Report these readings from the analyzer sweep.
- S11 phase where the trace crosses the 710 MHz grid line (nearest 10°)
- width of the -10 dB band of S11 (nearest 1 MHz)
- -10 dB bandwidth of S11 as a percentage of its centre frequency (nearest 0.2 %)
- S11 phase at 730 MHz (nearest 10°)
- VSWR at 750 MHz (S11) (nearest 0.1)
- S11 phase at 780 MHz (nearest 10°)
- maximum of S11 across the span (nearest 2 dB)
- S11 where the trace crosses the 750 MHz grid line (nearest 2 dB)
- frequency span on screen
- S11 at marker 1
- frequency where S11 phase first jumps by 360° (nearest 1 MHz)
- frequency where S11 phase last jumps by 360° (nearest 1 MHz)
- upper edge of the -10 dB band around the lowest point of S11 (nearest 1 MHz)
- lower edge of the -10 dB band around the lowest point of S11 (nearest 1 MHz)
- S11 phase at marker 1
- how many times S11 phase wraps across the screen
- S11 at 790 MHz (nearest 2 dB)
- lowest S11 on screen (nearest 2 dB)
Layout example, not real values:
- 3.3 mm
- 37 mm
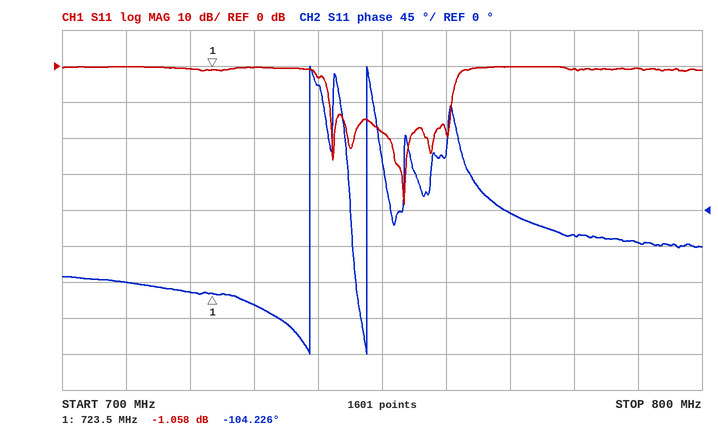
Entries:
- -90°
- 19 MHz
- 2.6 %
- -120°
- 1.3
- -30°
- 0 dB
- -18 dB
- 100 MHz
- -1.058 dB
- 739 MHz
- 748 MHz
- 761 MHz
- 742 MHz
- -104.226°
- 2
- 0 dB
- -38 dB
